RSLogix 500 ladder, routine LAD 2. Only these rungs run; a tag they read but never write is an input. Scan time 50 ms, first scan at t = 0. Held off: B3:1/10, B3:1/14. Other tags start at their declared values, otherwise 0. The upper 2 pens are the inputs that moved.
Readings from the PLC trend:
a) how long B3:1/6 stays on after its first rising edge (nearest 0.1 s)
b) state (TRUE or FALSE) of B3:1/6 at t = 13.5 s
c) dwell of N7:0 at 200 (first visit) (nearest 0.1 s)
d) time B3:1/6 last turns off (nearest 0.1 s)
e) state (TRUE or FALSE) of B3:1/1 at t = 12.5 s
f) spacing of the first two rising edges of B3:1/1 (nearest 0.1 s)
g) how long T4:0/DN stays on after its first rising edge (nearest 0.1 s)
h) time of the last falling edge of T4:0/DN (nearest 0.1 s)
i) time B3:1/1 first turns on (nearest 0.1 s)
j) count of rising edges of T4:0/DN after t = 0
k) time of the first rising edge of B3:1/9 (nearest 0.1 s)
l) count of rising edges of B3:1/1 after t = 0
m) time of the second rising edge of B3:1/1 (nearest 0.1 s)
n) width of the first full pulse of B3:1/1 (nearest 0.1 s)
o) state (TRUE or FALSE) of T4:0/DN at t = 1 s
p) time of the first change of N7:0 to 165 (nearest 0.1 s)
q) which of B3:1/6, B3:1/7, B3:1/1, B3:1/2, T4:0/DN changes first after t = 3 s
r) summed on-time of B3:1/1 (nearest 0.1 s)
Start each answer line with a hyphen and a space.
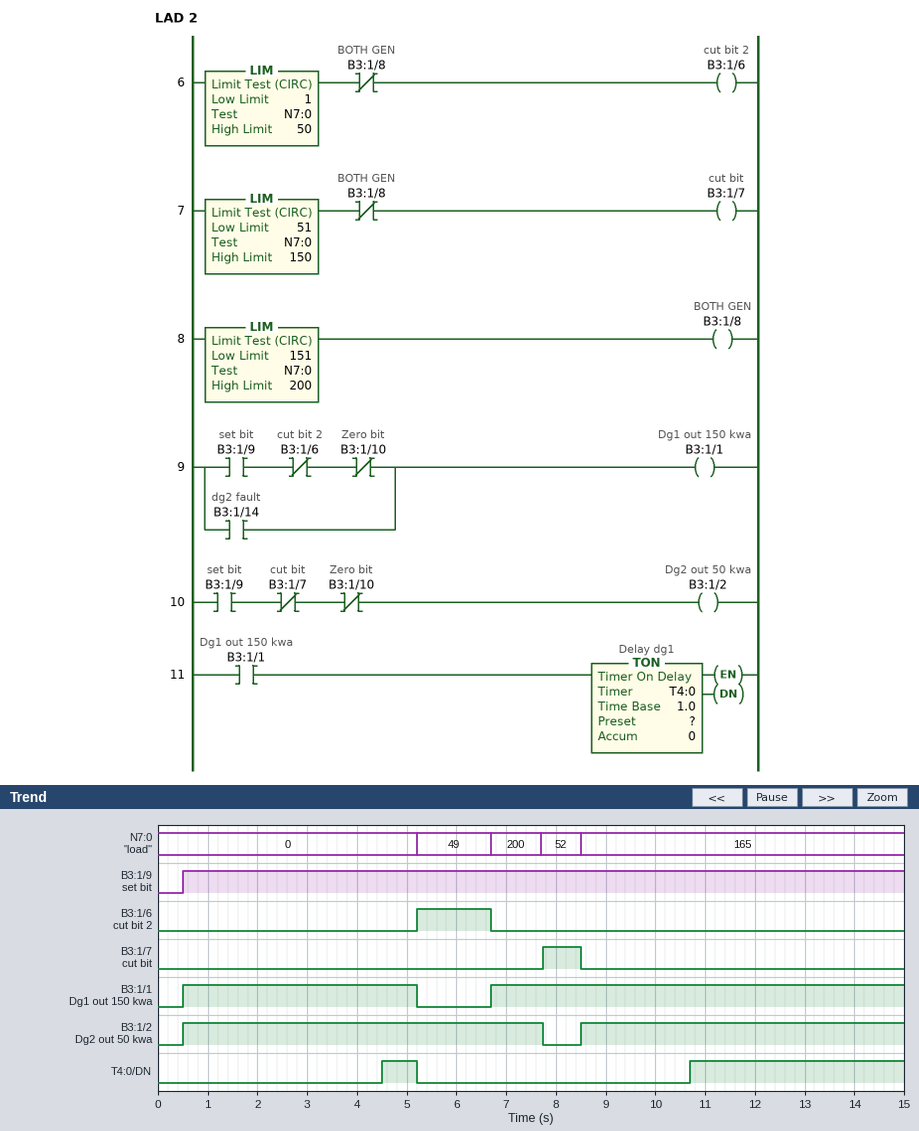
- 1.5 s
- FALSE
- 1.0 s
- 6.7 s
- TRUE
- 6.2 s
- 0.7 s
- 5.2 s
- 0.5 s
- 2
- 0.5 s
- 2
- 6.7 s
- 4.7 s
- FALSE
- 8.5 s
- T4:0/DN
- 13.0 s
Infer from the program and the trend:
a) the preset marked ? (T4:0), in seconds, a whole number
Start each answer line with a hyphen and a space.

- 4 s
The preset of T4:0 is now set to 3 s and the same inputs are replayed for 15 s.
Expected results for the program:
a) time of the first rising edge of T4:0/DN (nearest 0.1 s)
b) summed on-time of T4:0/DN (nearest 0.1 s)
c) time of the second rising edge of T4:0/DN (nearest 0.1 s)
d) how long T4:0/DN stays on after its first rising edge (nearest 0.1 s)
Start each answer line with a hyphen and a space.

- 3.5 s
- 7.0 s
- 9.7 s
- 1.7 s
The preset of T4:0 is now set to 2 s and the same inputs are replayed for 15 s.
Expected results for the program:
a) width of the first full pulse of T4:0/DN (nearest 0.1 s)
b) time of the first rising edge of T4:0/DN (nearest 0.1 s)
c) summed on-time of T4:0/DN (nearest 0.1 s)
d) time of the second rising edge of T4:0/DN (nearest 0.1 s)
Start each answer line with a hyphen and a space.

- 2.7 s
- 2.5 s
- 9.0 s
- 8.7 s
